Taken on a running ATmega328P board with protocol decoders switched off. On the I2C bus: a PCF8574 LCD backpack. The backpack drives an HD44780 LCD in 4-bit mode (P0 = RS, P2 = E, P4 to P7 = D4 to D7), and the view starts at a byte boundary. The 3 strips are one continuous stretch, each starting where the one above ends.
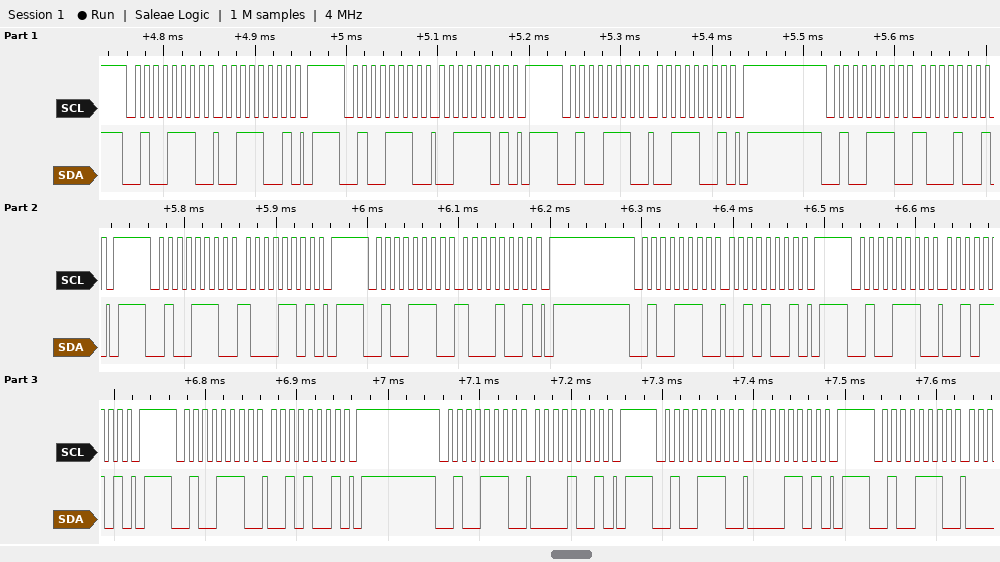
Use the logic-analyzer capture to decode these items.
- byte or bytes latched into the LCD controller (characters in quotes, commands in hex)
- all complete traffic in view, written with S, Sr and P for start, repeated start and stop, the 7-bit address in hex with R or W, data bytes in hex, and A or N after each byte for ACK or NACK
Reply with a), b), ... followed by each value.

a) '8'
b) S 27W A 39 A P S 27W A 3D A P S 27W A 39 A P S 27W A 89 A P S 27W A 8D A P S 27W A 89 A P S 27W A 29 A P S 27W A 2D A P S 27W A 29 A P S 27W A 09 A P S 27W A 0D A P S 27W A
